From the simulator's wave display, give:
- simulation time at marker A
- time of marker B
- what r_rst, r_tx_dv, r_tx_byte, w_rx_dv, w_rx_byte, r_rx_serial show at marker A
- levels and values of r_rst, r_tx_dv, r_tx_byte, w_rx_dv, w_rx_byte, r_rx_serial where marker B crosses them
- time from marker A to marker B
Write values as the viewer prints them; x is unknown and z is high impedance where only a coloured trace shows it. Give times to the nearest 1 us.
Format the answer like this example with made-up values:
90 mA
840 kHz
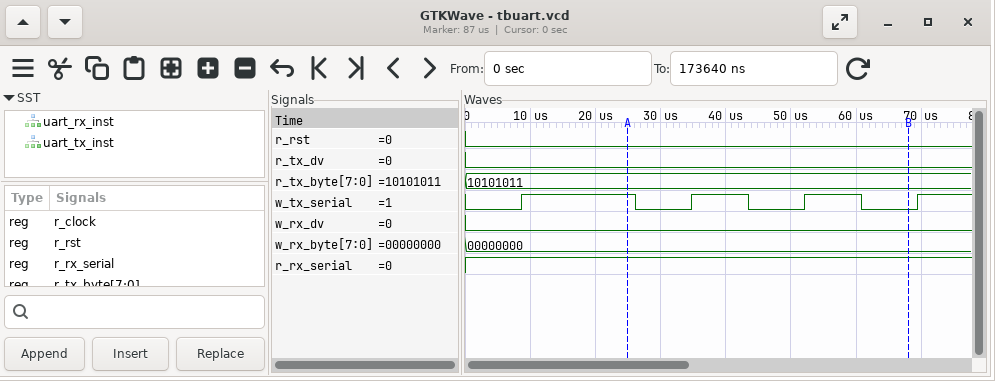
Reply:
25 us
68 us
r_rst=0, r_tx_dv=0, r_tx_byte=10101011, w_rx_dv=0, w_rx_byte=00000000, r_rx_serial=1
r_rst=0, r_tx_dv=0, r_tx_byte=10101011, w_rx_dv=0, w_rx_byte=00000000, r_rx_serial=1
43 us
